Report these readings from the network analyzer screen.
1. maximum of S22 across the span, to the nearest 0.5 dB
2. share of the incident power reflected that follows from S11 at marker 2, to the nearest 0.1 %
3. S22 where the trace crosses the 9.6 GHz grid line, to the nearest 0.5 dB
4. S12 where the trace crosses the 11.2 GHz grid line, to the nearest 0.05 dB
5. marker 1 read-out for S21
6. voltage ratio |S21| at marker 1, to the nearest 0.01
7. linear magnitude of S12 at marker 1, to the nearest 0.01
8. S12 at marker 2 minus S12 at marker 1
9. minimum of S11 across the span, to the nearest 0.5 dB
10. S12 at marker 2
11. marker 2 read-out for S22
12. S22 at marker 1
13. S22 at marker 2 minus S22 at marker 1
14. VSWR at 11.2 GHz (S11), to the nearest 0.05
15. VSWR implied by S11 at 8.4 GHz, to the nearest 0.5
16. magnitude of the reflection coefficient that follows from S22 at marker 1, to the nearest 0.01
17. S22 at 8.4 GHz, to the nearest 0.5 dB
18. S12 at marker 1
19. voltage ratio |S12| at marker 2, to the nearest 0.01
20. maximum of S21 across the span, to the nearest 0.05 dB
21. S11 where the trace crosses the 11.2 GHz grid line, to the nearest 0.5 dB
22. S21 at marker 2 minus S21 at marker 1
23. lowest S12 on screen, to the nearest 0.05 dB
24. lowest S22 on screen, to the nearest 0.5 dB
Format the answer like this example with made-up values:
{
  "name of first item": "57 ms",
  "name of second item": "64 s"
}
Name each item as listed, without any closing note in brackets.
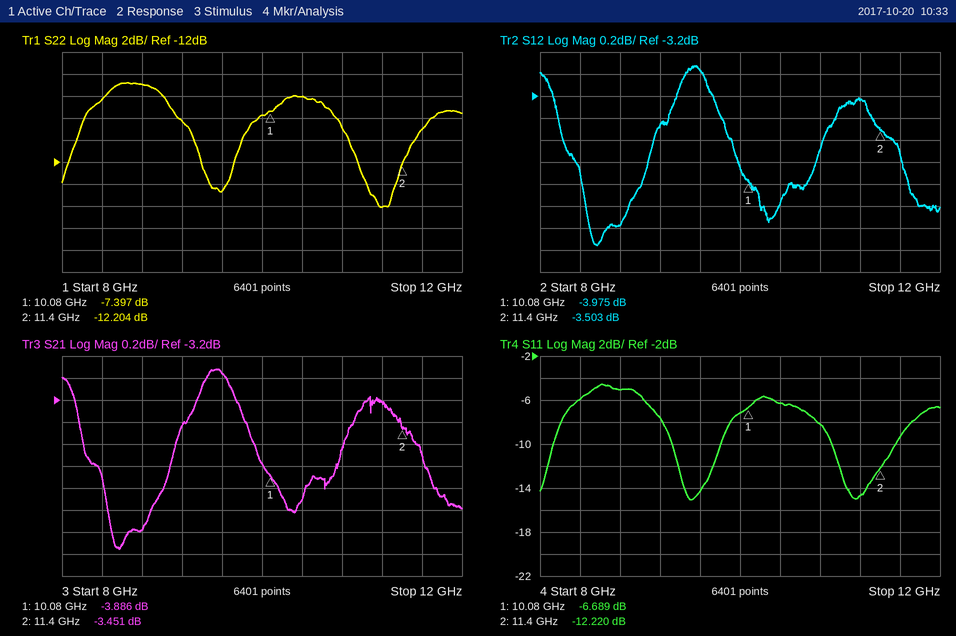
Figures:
{
  "maximum of S22 across the span, to the nearest 0.5 dB": "-5.0 dB",
  "share of the incident power reflected that follows from S11 at marker 2, to the nearest 0.1 %": "6.0 %",
  "S22 where the trace crosses the 9.6 GHz grid line, to the nearest 0.5 dB": "-14.5 dB",
  "S12 where the trace crosses the 11.2 GHz grid line, to the nearest 0.05 dB": "-3.25 dB",
  "marker 1 read-out for S21": "-3.886 dB",
  "voltage ratio |S21| at marker 1, to the nearest 0.01": "0.64",
  "linear magnitude of S12 at marker 1, to the nearest 0.01": "0.63",
  "S12 at marker 2 minus S12 at marker 1": "0.472 dB",
  "minimum of S11 across the span, to the nearest 0.5 dB": "-15.0 dB",
  "S12 at marker 2": "-3.503 dB",
  "marker 2 read-out for S22": "-12.204 dB",
  "S22 at marker 1": "-7.397 dB",
  "S22 at marker 2 minus S22 at marker 1": "-4.807 dB",
  "VSWR at 11.2 GHz (S11), to the nearest 0.05": "1.45",
  "VSWR implied by S11 at 8.4 GHz, to the nearest 0.5": "3.0",
  "magnitude of the reflection coefficient that follows from S22 at marker 1, to the nearest 0.01": "0.43",
  "S22 at 8.4 GHz, to the nearest 0.5 dB": "-6.5 dB",
  "S12 at marker 1": "-3.975 dB",
  "voltage ratio |S12| at marker 2, to the nearest 0.01": "0.67",
  "maximum of S21 across the span, to the nearest 0.05 dB": "-2.90 dB",
  "S11 where the trace crosses the 11.2 GHz grid line, to the nearest 0.5 dB": "-14.5 dB",
  "S21 at marker 2 minus S21 at marker 1": "0.435 dB",
  "lowest S12 on screen, to the nearest 0.05 dB": "-4.55 dB",
  "lowest S22 on screen, to the nearest 0.5 dB": "-16.0 dB"
}
